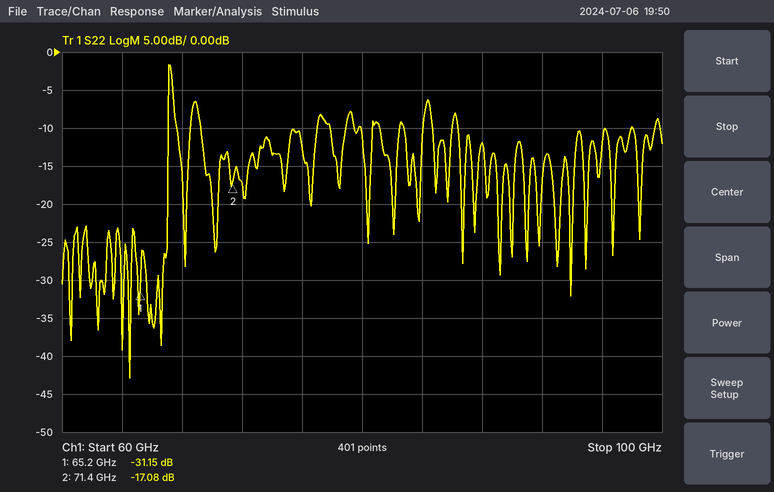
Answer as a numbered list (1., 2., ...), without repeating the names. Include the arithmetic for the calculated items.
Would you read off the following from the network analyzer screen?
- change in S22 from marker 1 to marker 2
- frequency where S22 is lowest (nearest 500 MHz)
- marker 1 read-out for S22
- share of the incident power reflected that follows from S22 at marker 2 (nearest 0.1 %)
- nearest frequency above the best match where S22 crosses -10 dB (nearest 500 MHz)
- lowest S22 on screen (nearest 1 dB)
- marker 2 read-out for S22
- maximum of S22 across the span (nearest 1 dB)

1. -17.08 − (-31.15) = 14.07 dB
2. 64.5 GHz
3. -31.15 dB
4. 10^(-17.08/10) ≈ 2.0 %
5. 67.0 GHz
6. -43 dB
7. -17.08 dB
8. -2 dB
